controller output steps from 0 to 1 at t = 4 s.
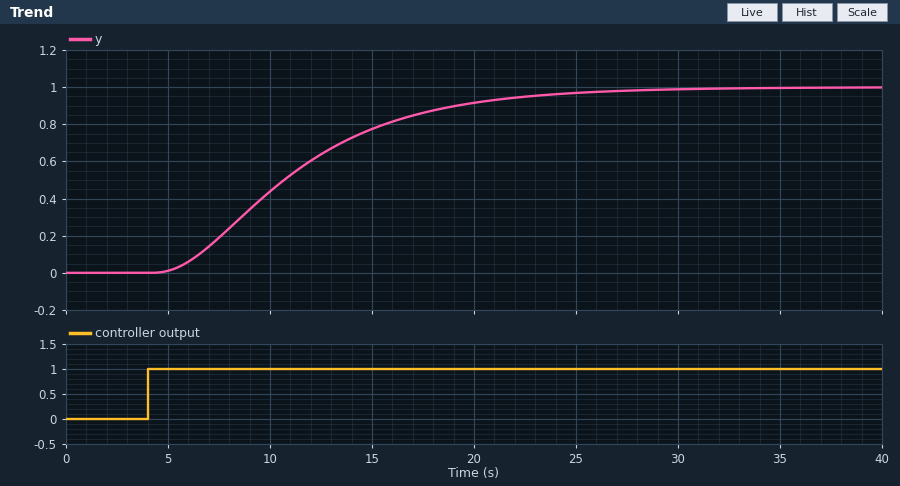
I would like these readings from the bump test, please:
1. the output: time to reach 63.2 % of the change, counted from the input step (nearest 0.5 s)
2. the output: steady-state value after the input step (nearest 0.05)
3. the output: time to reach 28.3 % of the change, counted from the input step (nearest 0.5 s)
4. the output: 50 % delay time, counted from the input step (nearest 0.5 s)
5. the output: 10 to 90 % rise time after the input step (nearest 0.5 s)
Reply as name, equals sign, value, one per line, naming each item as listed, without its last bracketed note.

the output: time to reach 63.2 % of the change, counted from the input step = 8.5 s
the output: steady-state value after the input step = 1.00
the output: time to reach 28.3 % of the change, counted from the input step = 4.5 s
the output: 50 % delay time, counted from the input step = 6.5 s
the output: 10 to 90 % rise time after the input step = 12.5 s
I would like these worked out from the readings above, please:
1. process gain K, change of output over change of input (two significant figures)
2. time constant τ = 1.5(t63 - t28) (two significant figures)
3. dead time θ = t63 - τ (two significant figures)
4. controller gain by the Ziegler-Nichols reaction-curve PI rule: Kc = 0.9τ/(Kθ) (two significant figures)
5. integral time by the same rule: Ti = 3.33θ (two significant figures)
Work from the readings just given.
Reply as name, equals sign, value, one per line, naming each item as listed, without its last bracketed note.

process gain K, change of output over change of input = 1.0
time constant τ = 1.5(t63 - t28) = 6.0 s
dead time θ = t63 - τ = 2.5 s
controller gain by the Ziegler-Nichols reaction-curve PI rule: Kc = 0.9τ/(Kθ) = 2.2
integral time by the same rule: Ti = 3.33θ = 8.3 s
